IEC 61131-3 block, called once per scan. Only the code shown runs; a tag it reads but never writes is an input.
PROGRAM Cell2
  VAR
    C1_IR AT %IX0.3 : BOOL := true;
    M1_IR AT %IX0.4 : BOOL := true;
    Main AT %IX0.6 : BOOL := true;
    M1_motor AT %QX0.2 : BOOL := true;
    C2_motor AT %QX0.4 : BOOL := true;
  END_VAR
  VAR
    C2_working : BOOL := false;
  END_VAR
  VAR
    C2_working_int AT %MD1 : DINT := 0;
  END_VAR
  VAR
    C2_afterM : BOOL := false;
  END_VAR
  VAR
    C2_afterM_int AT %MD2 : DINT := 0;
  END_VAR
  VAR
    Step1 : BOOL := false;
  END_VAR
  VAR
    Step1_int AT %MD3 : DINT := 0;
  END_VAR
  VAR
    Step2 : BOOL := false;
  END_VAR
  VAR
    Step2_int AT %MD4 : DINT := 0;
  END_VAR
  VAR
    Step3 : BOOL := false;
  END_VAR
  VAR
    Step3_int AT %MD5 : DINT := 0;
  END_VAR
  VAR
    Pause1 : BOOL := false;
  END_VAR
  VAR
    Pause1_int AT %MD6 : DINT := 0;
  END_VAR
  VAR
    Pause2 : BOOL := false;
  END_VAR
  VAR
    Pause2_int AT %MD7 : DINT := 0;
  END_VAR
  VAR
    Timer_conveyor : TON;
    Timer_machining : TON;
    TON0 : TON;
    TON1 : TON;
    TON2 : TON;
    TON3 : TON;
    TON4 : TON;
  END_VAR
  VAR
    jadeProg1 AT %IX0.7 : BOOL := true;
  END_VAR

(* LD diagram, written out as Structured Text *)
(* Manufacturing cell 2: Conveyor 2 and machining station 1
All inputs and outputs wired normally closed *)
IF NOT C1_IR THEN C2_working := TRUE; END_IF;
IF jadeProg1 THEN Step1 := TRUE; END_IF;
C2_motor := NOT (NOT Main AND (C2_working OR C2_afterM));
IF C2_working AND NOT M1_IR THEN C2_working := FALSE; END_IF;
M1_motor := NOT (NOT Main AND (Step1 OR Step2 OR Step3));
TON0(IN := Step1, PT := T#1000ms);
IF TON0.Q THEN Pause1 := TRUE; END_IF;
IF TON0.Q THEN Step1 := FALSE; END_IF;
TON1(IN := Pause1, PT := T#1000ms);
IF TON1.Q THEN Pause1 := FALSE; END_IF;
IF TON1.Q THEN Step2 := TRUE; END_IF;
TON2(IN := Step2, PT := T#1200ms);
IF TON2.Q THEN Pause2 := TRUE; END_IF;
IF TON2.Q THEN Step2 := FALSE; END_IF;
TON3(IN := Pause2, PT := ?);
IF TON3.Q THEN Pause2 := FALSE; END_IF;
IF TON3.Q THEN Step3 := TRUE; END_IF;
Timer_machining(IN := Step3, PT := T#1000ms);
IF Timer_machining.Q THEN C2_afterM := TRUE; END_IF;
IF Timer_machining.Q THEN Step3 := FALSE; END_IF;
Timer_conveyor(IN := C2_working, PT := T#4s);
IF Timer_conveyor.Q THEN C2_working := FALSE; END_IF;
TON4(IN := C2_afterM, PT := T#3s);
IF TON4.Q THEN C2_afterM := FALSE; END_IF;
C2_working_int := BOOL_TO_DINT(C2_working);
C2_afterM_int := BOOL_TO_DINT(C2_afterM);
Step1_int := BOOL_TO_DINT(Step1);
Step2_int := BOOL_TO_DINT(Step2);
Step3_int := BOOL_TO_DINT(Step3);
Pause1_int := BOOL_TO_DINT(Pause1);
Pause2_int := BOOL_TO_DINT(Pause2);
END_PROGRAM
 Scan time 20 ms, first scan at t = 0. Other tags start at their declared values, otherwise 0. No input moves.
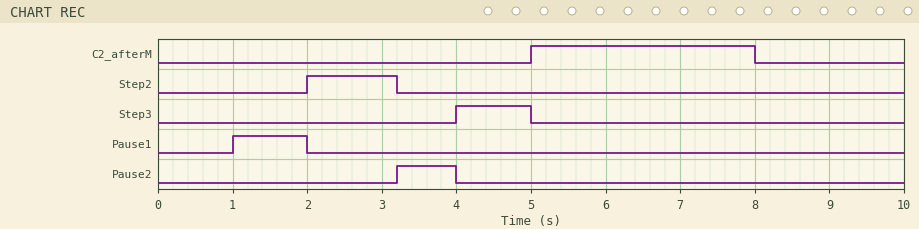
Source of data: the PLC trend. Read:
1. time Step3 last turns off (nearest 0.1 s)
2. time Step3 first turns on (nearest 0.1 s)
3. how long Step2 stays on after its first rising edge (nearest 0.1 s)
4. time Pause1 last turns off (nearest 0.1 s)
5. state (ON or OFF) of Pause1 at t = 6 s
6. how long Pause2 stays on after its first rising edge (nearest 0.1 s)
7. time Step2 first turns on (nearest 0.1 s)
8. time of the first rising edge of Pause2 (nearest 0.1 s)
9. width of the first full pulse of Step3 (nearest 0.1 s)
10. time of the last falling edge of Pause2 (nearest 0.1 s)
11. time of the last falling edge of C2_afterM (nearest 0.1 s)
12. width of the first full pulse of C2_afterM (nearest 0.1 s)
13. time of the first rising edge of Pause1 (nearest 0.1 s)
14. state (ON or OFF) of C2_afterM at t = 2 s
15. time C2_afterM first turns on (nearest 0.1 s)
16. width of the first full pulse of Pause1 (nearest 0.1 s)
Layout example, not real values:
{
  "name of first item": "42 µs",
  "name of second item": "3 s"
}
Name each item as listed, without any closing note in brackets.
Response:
{
  "time Step3 last turns off": "5.0 s",
  "time Step3 first turns on": "4.0 s",
  "how long Step2 stays on after its first rising edge": "1.2 s",
  "time Pause1 last turns off": "2.0 s",
  "state (ON or OFF) of Pause1 at t = 6 s": "OFF",
  "how long Pause2 stays on after its first rising edge": "0.8 s",
  "time Step2 first turns on": "2.0 s",
  "time of the first rising edge of Pause2": "3.2 s",
  "width of the first full pulse of Step3": "1.0 s",
  "time of the last falling edge of Pause2": "4.0 s",
  "time of the last falling edge of C2_afterM": "8.0 s",
  "width of the first full pulse of C2_afterM": "3.0 s",
  "time of the first rising edge of Pause1": "1.0 s",
  "state (ON or OFF) of C2_afterM at t = 2 s": "OFF",
  "time C2_afterM first turns on": "5.0 s",
  "width of the first full pulse of Pause1": "1.0 s"
}
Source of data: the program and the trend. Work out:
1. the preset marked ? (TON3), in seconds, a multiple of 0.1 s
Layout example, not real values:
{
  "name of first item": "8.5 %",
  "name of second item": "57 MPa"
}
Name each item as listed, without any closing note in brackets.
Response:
{
  "the preset marked ? (TON3), in seconds, a multiple of 0.1 s": "0.8 s"
}
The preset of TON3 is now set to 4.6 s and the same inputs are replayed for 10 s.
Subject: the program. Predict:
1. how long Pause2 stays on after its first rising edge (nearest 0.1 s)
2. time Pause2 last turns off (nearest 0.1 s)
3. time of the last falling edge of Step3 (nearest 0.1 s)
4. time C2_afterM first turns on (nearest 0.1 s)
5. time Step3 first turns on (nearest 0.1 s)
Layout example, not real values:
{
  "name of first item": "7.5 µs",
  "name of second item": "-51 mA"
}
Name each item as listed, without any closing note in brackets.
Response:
{
  "how long Pause2 stays on after its first rising edge": "4.6 s",
  "time Pause2 last turns off": "7.8 s",
  "time of the last falling edge of Step3": "8.8 s",
  "time C2_afterM first turns on": "8.8 s",
  "time Step3 first turns on": "7.8 s"
}
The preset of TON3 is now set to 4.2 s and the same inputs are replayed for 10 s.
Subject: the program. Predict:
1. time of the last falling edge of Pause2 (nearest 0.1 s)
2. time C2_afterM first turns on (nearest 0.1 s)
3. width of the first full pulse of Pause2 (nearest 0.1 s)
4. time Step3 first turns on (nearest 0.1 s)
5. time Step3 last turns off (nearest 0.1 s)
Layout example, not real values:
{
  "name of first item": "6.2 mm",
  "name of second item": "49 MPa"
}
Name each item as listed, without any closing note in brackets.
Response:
{
  "time of the last falling edge of Pause2": "7.4 s",
  "time C2_afterM first turns on": "8.4 s",
  "width of the first full pulse of Pause2": "4.2 s",
  "time Step3 first turns on": "7.4 s",
  "time Step3 last turns off": "8.4 s"
}
